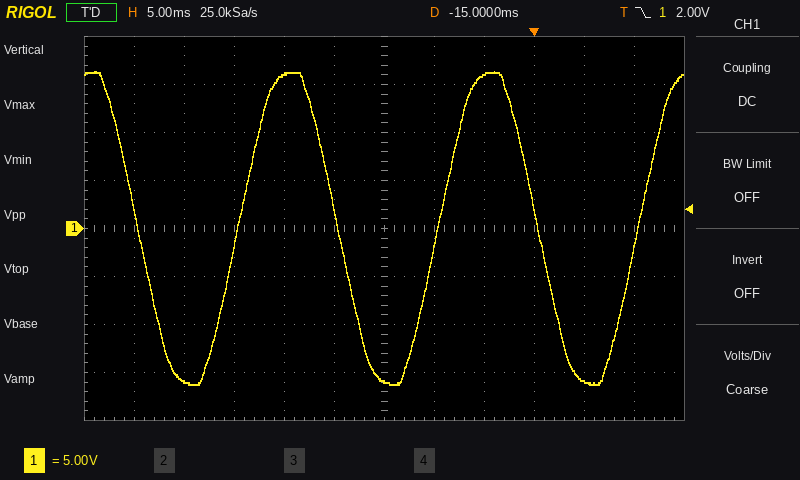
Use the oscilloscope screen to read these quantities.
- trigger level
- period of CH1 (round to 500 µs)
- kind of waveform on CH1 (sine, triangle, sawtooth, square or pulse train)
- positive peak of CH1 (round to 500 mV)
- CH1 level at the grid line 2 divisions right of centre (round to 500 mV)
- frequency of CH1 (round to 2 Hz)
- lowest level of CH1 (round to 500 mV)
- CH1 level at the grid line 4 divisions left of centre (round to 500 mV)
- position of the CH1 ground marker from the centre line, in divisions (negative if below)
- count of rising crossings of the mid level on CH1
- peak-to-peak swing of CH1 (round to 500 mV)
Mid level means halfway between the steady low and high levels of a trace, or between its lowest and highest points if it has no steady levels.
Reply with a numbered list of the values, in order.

1. 2.00 V
2. 20.0 ms
3. sine
4. 16.5 V
5. 16.0 V
6. 50 Hz
7. -16.0 V
8. -16.0 V
9. 0.0 div
10. 3
11. 32.5 V
